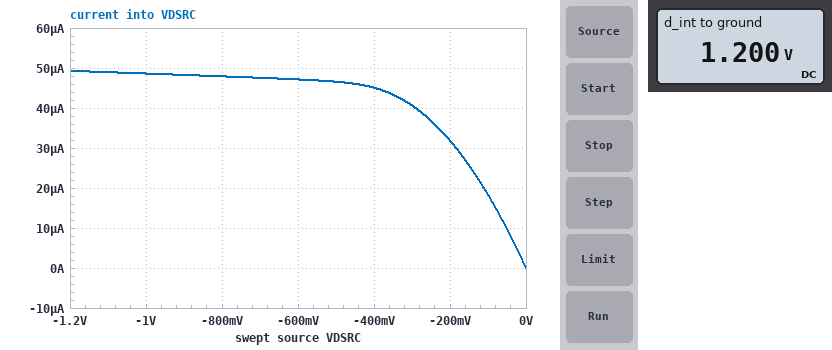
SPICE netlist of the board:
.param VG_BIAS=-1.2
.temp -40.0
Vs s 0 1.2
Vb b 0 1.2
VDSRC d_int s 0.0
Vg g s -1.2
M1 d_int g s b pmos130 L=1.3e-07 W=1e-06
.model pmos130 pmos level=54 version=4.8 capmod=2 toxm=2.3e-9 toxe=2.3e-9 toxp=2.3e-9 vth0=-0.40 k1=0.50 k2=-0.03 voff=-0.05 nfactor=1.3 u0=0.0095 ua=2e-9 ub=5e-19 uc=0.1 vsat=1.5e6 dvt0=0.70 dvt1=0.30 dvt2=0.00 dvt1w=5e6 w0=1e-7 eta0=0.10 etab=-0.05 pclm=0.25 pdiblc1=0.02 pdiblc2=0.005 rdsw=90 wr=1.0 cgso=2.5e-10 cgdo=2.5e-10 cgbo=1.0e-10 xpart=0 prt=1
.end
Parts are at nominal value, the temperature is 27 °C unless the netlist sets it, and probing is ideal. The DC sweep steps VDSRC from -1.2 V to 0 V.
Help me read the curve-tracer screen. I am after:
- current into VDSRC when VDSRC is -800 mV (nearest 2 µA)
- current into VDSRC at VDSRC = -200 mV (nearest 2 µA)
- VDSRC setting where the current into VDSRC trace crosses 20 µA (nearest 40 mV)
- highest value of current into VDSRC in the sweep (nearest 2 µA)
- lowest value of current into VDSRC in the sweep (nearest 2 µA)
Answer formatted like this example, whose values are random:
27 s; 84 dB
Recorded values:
48 µA; 32 µA; -120 mV; 50 µA; 0 A
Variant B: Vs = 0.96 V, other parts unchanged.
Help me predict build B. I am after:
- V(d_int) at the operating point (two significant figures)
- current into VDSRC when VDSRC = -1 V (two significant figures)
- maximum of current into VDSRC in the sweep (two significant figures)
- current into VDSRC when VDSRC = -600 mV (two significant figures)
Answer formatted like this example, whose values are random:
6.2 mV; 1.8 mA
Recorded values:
960 mV; 990 µA; 1.0 mA; 930 µA
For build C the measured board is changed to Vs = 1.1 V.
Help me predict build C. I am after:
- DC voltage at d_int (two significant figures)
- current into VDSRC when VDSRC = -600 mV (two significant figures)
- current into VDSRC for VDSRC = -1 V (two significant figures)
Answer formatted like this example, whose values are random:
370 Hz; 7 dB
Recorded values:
1.1 V; 1.0 mA; 1.1 mA
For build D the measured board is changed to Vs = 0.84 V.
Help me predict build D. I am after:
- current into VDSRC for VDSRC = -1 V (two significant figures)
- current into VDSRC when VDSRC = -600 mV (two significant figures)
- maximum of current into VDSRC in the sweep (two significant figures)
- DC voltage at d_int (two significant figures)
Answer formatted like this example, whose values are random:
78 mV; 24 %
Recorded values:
910 µA; 850 µA; 930 µA; 840 mV
